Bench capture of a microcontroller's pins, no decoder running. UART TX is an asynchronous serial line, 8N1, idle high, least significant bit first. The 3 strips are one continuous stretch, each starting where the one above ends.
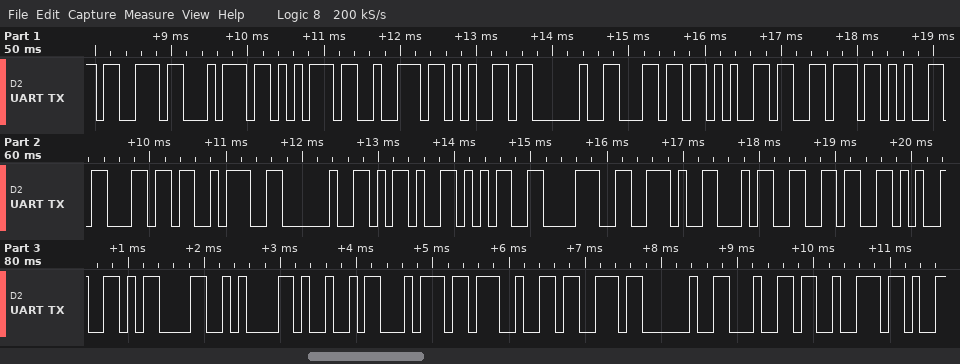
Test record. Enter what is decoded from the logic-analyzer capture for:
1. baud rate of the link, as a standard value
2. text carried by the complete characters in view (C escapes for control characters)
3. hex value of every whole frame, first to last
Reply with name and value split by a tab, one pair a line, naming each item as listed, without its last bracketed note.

baud rate of the link, as a standard value	9600 baud
text carried by the complete characters in view	"sture level: -58.46%\r\nIt's dr"
hex value of every whole frame, first to last	73 74 75 72 65 20 6C 65 76 65 6C 3A 20 2D 35 38 2E 34 36 25 0D 0A 49 74 27 73 20 64 72
